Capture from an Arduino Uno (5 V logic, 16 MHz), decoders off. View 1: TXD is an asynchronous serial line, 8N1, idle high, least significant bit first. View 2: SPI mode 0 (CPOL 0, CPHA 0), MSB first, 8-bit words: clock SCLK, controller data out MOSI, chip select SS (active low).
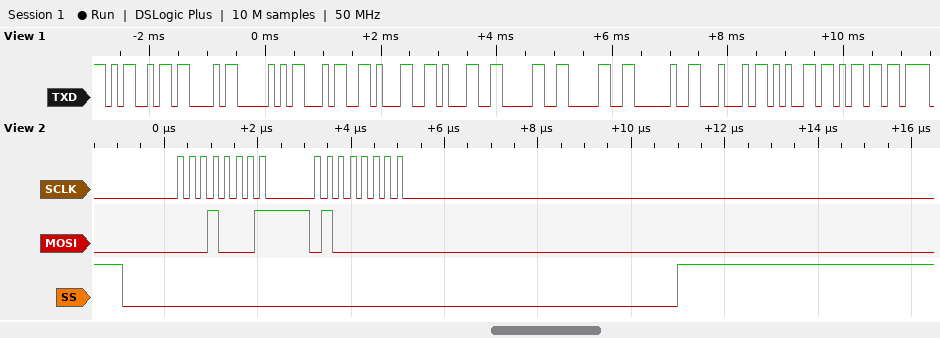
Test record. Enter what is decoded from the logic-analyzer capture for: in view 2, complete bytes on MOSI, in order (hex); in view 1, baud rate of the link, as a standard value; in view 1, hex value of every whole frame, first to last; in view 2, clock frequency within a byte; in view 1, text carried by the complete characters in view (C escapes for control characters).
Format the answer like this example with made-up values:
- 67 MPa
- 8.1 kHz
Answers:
- 11 40
- 9600 baud
- 4D 43 50 34 31 31 30 30 20 44 65 6D
- 4 MHz
- "MCP41100 Dem"
